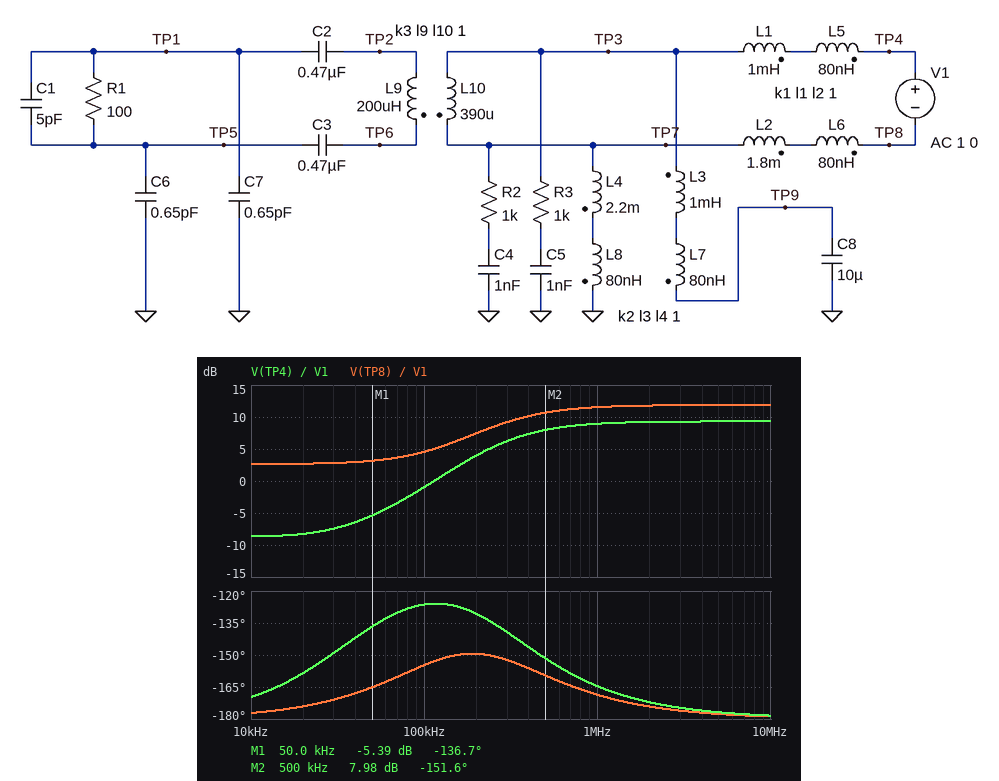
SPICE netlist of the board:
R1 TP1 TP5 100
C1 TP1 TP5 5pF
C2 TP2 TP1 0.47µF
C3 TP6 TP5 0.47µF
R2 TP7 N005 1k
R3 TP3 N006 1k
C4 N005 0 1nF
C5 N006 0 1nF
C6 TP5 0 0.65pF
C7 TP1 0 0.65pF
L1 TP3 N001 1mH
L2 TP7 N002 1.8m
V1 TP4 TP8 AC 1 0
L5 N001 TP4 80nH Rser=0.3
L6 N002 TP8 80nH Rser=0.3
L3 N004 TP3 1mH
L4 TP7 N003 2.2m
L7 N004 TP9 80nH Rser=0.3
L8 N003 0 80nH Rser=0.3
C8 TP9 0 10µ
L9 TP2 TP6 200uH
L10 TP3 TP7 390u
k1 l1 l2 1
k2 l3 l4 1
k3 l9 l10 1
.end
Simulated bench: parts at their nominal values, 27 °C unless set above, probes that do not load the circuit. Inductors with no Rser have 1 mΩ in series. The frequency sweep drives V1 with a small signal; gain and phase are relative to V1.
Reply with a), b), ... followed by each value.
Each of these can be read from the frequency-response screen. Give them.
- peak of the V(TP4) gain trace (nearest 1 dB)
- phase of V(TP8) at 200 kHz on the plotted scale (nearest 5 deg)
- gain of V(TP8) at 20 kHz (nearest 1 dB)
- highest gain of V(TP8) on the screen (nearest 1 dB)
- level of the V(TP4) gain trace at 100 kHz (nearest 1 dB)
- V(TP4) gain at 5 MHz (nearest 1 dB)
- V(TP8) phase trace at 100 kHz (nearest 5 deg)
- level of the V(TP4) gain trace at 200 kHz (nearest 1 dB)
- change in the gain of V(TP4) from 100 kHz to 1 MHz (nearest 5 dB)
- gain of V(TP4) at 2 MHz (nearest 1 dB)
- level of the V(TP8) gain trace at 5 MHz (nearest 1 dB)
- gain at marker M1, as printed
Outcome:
a) 9 dB
b) -150 deg
c) 3 dB
d) 12 dB
e) -1 dB
f) 9 dB
g) -155 deg
h) 4 dB
i) 10 dB
j) 9 dB
k) 12 dB
l) -5.39 dB
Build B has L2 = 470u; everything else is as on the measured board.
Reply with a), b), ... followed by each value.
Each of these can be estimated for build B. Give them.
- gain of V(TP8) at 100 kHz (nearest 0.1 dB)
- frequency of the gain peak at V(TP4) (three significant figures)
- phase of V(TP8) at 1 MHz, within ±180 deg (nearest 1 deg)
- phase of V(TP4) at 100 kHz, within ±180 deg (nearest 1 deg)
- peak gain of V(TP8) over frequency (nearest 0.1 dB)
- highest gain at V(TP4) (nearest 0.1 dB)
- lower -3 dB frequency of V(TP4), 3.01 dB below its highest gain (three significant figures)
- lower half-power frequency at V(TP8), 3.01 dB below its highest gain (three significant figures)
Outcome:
a) -5.0 dB
b) 634 Hz
c) 20 deg
d) 27 deg
e) 21.0 dB
f) 21.3 dB
g) 621 Hz
h) 623 Hz
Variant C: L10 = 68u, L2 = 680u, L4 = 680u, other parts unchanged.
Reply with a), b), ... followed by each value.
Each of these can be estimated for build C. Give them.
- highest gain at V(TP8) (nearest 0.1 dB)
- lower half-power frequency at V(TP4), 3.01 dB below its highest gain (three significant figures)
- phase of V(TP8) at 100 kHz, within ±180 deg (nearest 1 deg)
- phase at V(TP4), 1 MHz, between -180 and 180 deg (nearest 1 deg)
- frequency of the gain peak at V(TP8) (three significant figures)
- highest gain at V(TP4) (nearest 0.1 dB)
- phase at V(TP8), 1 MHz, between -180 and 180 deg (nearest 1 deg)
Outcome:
a) 13.6 dB
b) 838 Hz
c) 39 deg
d) 9 deg
e) 863 Hz
f) 15.2 dB
g) 11 deg
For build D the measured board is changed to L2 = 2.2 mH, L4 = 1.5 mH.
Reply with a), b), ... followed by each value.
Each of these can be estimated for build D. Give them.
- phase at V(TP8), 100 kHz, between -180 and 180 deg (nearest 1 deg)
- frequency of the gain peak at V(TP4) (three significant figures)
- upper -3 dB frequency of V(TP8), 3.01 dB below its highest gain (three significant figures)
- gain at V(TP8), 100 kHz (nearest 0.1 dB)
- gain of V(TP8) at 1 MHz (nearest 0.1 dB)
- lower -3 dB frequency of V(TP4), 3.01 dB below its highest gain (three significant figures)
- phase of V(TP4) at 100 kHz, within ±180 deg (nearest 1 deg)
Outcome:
a) -160 deg
b) 705 Hz
c) 721 Hz
d) 5.5 dB
e) 9.6 dB
f) 692 Hz
g) -140 deg
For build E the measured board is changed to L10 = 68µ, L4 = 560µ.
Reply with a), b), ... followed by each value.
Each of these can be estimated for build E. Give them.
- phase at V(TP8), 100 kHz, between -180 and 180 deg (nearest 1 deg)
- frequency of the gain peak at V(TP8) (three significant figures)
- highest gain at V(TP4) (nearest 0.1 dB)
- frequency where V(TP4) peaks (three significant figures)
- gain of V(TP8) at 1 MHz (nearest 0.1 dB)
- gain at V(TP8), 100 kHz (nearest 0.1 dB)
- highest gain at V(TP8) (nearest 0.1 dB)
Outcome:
a) -168 deg
b) 912 Hz
c) 13.2 dB
d) 908 Hz
e) 11.8 dB
f) 10.1 dB
g) 13.6 dB
